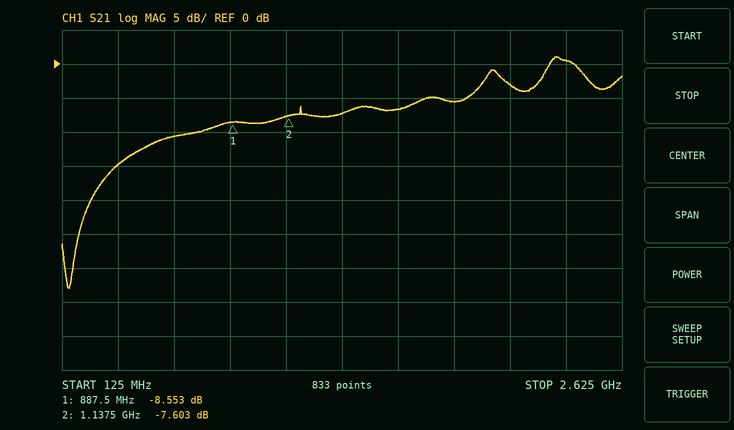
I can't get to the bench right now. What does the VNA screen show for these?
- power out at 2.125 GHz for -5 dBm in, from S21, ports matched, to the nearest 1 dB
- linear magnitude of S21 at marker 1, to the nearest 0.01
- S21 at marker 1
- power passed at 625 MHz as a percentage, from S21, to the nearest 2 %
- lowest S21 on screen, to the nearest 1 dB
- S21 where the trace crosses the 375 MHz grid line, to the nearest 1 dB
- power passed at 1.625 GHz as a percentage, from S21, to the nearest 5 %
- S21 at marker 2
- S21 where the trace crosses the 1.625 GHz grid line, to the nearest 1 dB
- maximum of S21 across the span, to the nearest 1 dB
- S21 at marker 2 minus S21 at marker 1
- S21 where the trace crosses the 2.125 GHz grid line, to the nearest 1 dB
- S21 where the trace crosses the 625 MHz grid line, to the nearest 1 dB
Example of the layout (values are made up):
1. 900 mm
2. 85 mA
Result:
1. -8 dBm
2. 0.37
3. -8.553 dB
4. 8 %
5. -33 dB
6. -15 dB
7. 20 %
8. -7.603 dB
9. -7 dB
10. 1 dB
11. 0.950 dB
12. -3 dB
13. -11 dB
